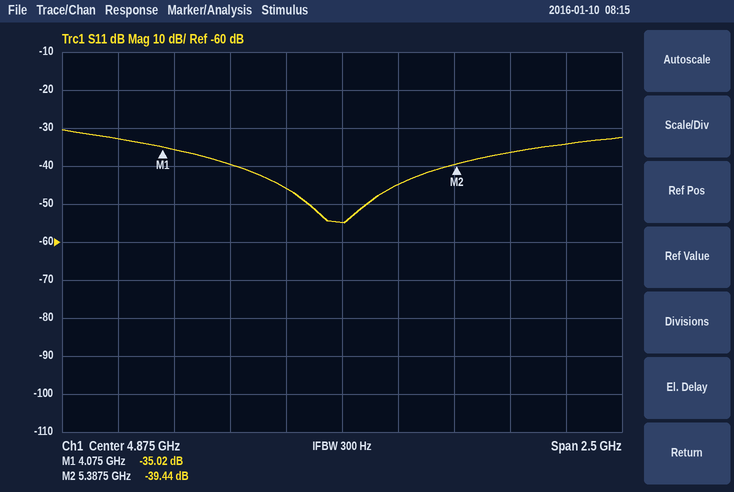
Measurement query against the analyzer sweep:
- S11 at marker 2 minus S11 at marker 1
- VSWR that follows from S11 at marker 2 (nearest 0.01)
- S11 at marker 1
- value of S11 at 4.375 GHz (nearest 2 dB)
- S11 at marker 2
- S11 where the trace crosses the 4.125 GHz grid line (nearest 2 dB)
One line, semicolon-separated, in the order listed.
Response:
-4.42 dB; 1.02; -35.02 dB; -40 dB; -39.44 dB; -36 dB
